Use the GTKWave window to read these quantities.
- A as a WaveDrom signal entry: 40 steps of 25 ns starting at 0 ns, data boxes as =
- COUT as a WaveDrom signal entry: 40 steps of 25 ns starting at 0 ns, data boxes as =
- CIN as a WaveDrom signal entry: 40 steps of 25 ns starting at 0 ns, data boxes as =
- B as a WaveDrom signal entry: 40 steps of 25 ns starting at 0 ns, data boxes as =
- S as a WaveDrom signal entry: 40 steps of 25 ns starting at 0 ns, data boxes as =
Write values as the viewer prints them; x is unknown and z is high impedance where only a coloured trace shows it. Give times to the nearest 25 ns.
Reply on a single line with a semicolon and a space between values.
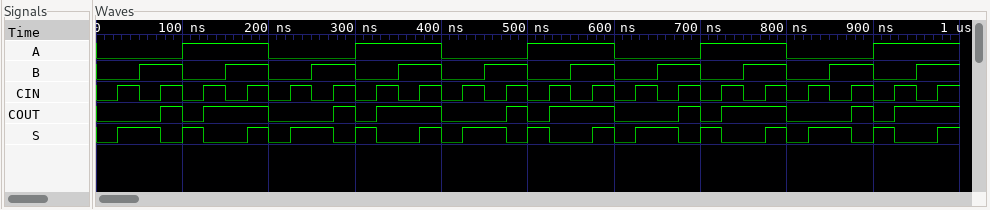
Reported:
{name: 'A', wave: '0...1...0...1...0...1...0...1...0...1...'}; {name: 'COUT', wave: '0..101..0..101..0..101..0..101..0..101..'}; {name: 'CIN', wave: '0101010101010101010101010101010101010101'}; {name: 'B', wave: '0.1.0.1.0.1.0.1.0.1.0.1.0.1.0.1.0.1.0.1.'}; {name: 'S', wave: '01.010.101.010.101.010.101.010.101.010.1'}
